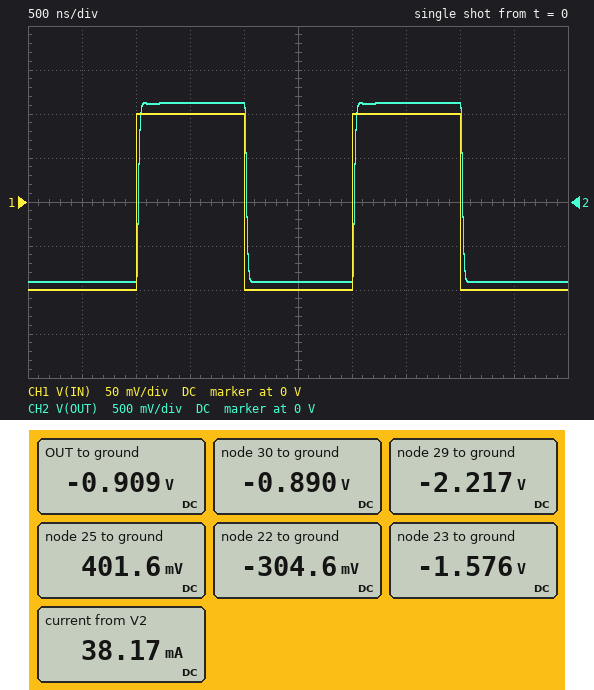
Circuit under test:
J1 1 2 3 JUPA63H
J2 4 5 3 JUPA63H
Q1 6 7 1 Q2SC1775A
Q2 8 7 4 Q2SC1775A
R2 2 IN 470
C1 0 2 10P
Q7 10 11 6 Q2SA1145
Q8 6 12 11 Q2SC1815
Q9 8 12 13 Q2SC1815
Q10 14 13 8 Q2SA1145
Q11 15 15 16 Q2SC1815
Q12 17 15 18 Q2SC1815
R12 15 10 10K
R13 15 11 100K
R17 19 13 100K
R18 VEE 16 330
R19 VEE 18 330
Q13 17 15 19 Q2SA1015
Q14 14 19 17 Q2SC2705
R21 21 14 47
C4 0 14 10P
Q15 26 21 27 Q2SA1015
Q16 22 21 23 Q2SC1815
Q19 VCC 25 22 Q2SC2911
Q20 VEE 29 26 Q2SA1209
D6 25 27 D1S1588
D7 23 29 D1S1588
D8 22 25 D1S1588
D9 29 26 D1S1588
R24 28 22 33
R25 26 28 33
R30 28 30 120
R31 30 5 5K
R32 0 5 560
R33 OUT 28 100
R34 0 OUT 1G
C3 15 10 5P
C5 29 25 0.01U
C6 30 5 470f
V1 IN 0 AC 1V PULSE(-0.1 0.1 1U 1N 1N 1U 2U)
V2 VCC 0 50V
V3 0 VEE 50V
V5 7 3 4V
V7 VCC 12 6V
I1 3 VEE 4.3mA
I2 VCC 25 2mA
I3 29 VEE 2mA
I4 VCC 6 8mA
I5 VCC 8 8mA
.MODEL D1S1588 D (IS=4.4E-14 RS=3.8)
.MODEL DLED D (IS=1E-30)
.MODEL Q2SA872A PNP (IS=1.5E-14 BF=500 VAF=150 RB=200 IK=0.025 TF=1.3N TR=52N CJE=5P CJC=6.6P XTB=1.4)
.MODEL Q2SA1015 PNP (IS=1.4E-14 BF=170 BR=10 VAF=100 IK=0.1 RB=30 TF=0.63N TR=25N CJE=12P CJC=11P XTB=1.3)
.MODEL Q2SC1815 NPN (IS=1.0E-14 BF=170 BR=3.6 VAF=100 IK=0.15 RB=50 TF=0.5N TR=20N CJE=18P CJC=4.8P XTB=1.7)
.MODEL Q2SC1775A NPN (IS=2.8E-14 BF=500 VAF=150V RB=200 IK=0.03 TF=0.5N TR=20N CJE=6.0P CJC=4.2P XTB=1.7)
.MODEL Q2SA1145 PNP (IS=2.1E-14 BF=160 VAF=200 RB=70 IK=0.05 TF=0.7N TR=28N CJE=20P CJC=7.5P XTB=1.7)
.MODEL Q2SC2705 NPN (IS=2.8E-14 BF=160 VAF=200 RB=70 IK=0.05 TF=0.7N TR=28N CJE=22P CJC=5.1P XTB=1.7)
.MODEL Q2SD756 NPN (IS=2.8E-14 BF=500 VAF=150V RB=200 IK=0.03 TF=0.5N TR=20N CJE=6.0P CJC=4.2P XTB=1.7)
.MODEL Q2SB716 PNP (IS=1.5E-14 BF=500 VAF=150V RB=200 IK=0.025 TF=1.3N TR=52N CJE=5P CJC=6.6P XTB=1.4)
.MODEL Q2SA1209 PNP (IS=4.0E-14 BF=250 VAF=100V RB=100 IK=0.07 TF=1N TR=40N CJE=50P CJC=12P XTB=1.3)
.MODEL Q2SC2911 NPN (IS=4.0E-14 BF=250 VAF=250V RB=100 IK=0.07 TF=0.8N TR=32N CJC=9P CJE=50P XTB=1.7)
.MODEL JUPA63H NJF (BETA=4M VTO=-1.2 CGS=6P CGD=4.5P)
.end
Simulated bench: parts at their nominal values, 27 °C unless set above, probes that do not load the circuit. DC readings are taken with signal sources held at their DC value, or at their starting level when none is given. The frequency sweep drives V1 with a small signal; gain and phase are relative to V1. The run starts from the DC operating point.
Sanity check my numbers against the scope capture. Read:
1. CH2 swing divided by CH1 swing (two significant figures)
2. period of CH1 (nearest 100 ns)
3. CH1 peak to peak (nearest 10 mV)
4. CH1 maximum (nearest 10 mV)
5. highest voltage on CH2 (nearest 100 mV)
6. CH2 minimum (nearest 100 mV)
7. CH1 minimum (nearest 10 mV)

10
2.0 µs
200 mV
100 mV
1.1 V
-900 mV
-100 mV
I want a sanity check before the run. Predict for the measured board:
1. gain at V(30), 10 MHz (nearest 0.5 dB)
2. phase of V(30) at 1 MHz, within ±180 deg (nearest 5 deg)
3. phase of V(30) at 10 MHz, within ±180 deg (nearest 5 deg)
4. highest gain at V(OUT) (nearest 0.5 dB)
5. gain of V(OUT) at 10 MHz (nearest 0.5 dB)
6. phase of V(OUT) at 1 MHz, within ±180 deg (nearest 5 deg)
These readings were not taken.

18.0 dB
-10 deg
-85 deg
20.0 dB
18.0 dB
-10 deg
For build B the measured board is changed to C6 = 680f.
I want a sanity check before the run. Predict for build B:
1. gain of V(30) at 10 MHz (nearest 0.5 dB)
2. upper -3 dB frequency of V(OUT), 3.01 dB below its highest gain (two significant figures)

17.5 dB
11 MHz
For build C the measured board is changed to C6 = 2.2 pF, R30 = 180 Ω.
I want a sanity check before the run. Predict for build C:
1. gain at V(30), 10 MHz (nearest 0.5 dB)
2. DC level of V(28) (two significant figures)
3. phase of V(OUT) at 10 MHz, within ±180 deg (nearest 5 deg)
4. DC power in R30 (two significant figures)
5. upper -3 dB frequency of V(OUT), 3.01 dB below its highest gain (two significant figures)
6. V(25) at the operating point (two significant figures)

15.0 dB
-920 mV
-90 deg
4.6 µW
7.0 MHz
390 mV
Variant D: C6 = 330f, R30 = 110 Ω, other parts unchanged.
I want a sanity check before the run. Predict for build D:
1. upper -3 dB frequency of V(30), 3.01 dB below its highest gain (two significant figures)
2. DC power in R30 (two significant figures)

13 MHz
2.8 µW
